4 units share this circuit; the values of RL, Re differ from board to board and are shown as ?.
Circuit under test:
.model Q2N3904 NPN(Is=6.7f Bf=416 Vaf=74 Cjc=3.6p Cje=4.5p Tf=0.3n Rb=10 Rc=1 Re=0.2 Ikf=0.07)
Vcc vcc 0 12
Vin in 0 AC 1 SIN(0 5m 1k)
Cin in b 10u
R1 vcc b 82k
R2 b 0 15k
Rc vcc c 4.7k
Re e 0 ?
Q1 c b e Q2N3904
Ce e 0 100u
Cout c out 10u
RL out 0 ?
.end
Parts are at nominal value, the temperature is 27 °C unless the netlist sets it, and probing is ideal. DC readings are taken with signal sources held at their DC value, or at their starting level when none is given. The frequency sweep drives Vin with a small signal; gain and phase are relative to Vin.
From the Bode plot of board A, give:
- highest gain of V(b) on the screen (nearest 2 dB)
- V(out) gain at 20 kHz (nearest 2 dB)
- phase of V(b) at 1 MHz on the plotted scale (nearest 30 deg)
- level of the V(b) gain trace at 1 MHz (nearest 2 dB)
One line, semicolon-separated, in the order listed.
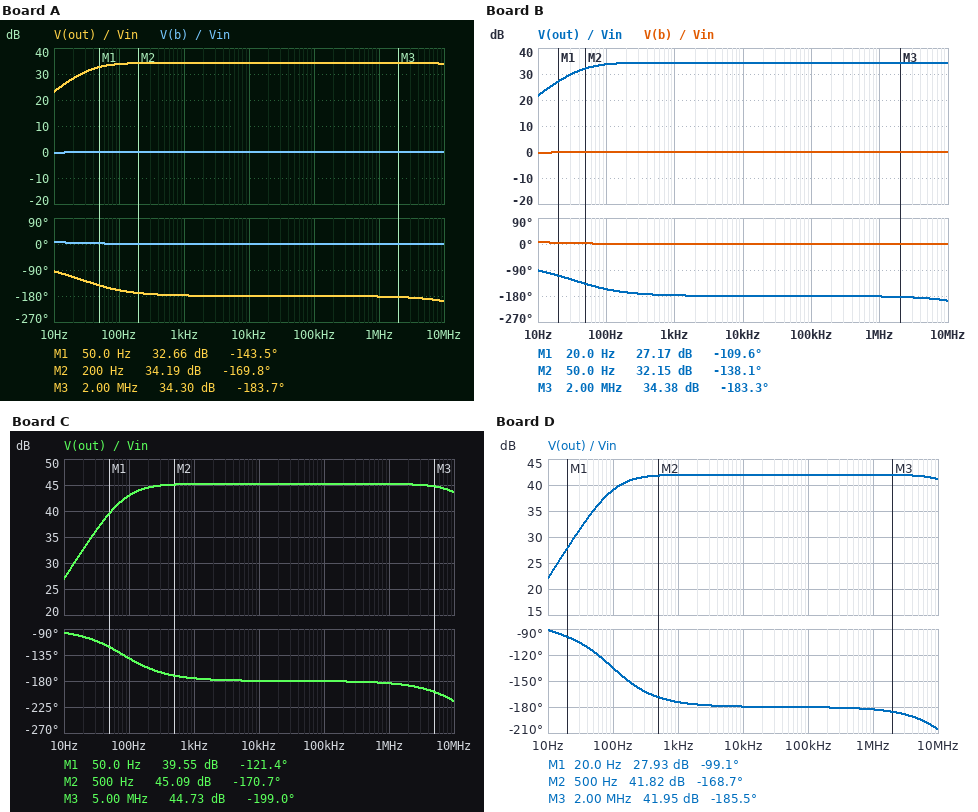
0 dB; 34 dB; 0 deg; 0 dB
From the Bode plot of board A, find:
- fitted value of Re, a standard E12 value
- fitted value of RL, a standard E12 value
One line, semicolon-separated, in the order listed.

2.2 kΩ; 5.6 kΩ
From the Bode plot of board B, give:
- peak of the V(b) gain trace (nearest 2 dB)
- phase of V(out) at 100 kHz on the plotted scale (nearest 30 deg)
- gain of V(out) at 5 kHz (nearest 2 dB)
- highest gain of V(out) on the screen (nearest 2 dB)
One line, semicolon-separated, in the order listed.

0 dB; -180 deg; 34 dB; 34 dB
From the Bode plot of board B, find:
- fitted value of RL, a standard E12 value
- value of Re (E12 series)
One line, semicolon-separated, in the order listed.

3.9 kΩ; 1.8 kΩ
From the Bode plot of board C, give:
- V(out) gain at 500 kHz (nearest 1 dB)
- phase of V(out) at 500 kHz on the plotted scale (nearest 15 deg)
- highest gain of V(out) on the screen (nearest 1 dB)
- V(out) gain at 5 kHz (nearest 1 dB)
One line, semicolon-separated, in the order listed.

45 dB; -180 deg; 45 dB; 45 dB
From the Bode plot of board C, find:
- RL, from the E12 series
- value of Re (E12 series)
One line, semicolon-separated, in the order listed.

18 kΩ; 820 Ω
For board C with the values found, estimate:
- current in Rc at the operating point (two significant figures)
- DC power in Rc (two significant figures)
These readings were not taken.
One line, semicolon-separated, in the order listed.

1.4 mA; 9.1 mW
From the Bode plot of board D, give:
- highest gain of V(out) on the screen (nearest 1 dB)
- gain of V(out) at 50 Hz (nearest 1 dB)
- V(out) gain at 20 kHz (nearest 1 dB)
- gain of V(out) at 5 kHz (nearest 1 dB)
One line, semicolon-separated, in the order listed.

42 dB; 35 dB; 42 dB; 42 dB
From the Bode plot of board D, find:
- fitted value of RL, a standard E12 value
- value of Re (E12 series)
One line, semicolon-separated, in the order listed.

3.9 kΩ; 680 Ω
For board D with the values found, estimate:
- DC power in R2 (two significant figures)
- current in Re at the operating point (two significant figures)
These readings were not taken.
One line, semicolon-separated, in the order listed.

220 µW; 1.7 mA
